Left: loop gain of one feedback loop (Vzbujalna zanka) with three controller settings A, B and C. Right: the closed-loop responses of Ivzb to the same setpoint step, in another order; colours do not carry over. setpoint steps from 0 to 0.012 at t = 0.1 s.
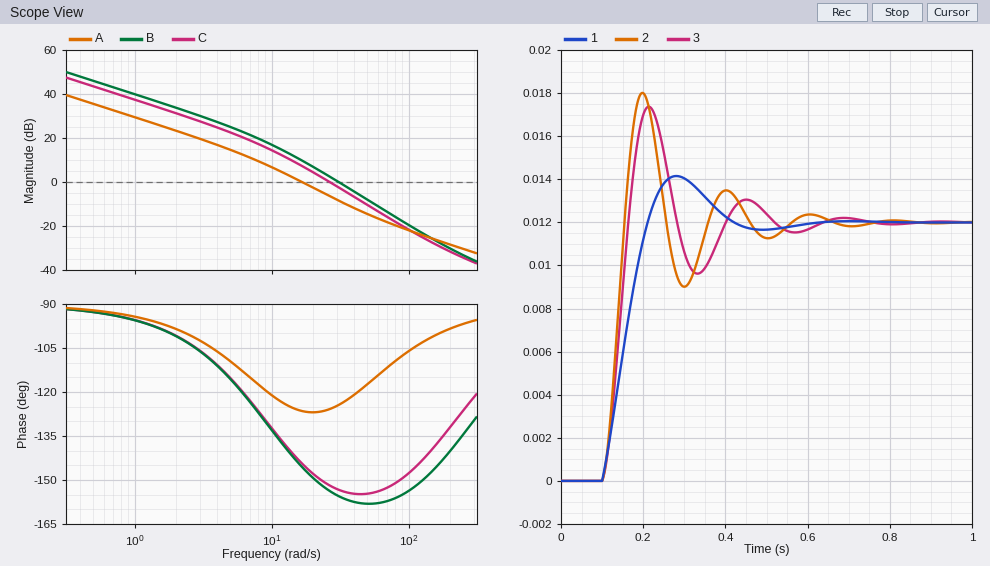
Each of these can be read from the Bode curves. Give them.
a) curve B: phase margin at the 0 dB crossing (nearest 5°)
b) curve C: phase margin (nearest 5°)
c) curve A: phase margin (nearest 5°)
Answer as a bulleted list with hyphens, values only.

- 25°
- 30°
- 55°
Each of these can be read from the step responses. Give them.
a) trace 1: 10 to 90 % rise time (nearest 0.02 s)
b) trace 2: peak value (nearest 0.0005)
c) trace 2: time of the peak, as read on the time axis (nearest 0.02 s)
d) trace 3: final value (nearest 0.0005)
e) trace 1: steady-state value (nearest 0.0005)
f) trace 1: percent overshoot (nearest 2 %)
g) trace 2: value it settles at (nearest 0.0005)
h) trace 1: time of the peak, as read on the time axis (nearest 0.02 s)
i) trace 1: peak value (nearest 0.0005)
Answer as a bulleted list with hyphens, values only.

- 0.08 s
- 0.0180
- 0.20 s
- 0.0120
- 0.0120
- 18 %
- 0.0120
- 0.28 s
- 0.0140
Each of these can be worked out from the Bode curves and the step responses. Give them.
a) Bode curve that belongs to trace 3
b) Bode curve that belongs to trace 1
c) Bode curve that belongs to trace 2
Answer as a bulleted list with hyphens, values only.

- C
- A
- B
